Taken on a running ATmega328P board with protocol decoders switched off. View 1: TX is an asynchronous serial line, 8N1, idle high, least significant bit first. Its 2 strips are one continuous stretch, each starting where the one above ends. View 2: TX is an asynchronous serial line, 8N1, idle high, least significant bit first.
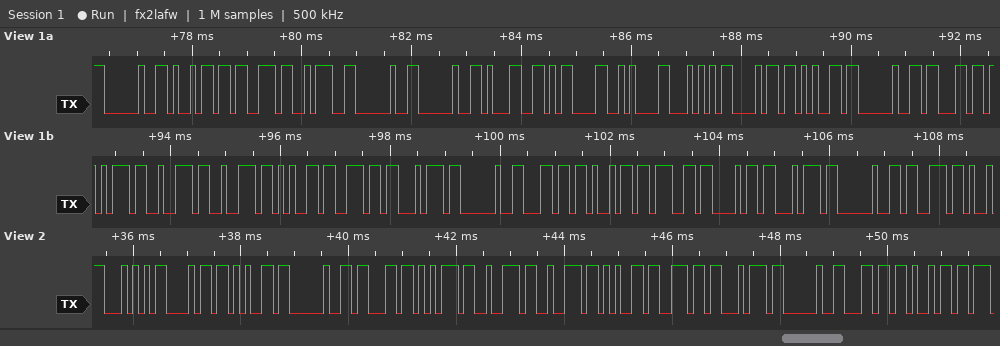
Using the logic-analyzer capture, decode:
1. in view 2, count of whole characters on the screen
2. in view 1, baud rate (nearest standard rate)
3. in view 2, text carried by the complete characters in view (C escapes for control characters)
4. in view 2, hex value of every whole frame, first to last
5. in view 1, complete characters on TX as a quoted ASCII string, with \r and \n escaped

14
9600 baud
"The current li"
54 68 65 20 63 75 72 72 65 6E 74 20 6C 69
" is:  1\r\nThe current light s"
